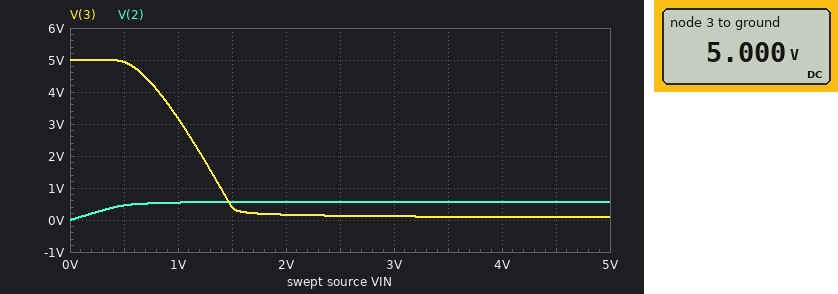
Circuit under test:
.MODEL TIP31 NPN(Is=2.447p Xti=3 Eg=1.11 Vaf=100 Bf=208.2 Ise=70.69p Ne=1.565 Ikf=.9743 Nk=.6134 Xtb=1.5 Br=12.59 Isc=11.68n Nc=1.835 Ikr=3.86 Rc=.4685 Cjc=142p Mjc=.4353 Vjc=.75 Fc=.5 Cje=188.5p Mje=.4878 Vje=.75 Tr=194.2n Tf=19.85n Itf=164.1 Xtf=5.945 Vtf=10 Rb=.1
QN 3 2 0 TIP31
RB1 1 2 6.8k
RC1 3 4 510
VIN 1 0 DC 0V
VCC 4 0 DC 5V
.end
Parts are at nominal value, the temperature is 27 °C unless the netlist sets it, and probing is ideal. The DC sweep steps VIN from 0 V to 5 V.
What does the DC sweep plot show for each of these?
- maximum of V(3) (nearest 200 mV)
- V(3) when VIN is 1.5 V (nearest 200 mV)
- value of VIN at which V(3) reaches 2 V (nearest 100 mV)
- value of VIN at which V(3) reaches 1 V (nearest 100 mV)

5.0 V
400 mV
1.2 V
1.4 V
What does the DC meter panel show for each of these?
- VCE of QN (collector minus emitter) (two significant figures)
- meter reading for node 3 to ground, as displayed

5.0 V
5.000 V
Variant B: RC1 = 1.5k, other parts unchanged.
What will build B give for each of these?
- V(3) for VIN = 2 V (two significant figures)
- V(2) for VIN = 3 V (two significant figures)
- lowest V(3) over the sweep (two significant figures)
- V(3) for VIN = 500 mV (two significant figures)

100 mV
550 mV
48 mV
4.8 V
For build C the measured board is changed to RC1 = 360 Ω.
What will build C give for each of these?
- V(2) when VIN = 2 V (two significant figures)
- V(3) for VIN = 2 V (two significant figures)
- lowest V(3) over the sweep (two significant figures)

580 mV
220 mV
93 mV
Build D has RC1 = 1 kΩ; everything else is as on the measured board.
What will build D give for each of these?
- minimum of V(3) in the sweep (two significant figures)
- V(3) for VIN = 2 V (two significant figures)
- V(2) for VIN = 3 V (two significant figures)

58 mV
120 mV
560 mV
